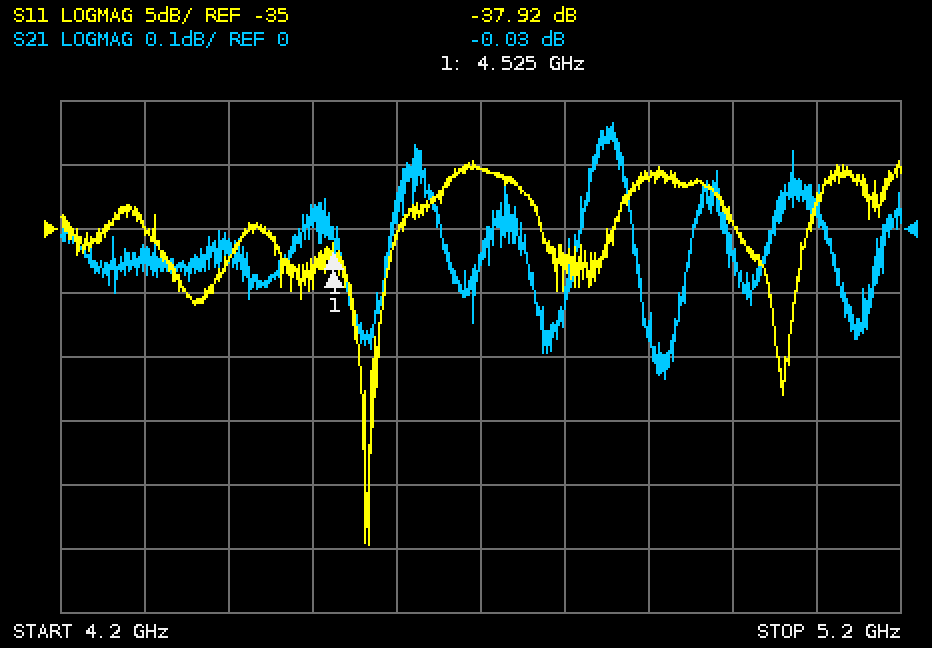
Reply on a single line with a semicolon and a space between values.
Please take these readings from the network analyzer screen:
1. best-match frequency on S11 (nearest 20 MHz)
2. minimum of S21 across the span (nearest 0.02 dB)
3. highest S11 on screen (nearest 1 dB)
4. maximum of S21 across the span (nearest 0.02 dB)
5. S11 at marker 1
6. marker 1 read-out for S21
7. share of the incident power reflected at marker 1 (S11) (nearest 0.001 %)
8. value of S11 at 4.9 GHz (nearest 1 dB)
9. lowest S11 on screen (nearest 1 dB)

4.56 GHz; -0.24 dB; -30 dB; 0.16 dB; -37.92 dB; -0.03 dB; 0.016 %; -31 dB; -60 dB
